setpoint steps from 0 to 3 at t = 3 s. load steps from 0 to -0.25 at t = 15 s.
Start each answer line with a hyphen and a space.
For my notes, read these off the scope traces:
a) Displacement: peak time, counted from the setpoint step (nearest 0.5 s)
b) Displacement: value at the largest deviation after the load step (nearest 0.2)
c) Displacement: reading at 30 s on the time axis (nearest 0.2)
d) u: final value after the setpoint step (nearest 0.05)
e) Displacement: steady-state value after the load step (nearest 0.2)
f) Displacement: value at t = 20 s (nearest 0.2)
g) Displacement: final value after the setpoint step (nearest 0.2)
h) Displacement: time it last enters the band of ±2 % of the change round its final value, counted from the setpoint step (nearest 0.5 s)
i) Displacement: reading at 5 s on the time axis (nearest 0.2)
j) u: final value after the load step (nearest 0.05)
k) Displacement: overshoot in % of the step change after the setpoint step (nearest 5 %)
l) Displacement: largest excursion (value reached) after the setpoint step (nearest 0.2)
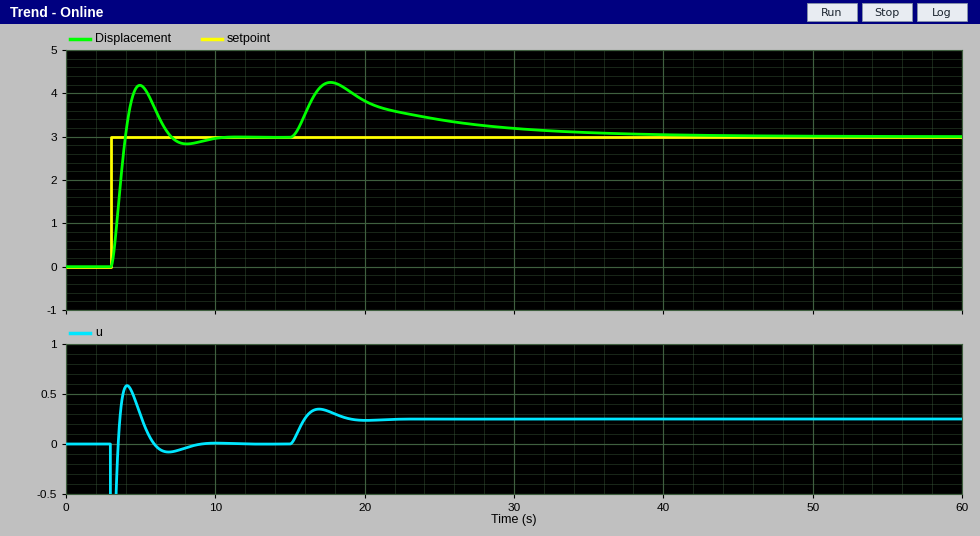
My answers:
- 2.0 s
- 4.2
- 3.2
- 0.00
- 3.0
- 3.8
- 3.0
- 6.5 s
- 4.2
- 0.25
- 40 %
- 4.2
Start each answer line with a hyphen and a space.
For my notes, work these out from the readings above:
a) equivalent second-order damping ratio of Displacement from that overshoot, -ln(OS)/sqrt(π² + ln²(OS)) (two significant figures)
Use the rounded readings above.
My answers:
- 0.28
